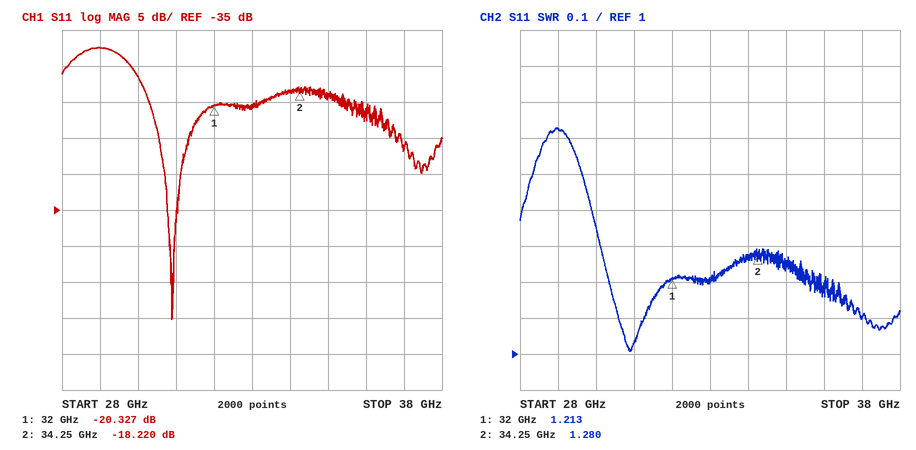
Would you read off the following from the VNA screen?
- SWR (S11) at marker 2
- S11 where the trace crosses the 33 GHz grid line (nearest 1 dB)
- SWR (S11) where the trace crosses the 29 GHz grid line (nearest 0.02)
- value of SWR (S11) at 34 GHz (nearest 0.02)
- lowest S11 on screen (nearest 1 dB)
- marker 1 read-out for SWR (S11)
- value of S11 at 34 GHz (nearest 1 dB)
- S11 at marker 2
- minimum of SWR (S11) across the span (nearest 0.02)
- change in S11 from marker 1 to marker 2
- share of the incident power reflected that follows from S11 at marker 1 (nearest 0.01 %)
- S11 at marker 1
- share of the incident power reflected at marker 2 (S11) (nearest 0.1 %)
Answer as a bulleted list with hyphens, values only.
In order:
- 1.280
- -21 dB
- 1.62
- 1.26
- -50 dB
- 1.213
- -19 dB
- -18.220 dB
- 1.00
- 2.107 dB
- 0.93 %
- -20.327 dB
- 1.5 %
